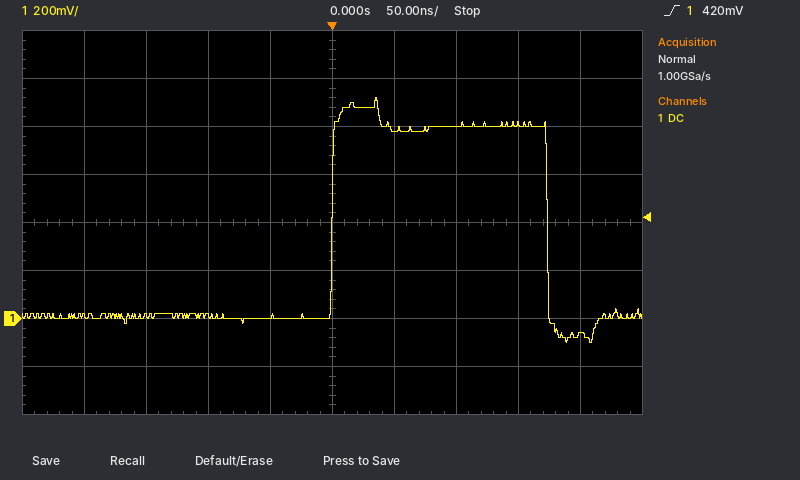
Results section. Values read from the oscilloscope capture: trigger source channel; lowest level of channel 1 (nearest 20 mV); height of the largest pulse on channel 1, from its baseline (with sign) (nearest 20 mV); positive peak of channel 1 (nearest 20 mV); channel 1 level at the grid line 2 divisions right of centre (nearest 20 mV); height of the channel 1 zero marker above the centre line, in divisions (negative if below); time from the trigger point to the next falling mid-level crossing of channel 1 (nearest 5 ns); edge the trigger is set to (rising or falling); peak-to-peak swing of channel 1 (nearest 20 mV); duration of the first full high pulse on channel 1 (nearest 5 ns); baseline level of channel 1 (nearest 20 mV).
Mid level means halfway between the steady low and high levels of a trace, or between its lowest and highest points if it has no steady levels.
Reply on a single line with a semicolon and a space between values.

channel 1; -100 mV; +920 mV; 920 mV; 800 mV; -2.0 div; 175 ns; rising; 1.02 V; 175 ns; 0 mV
